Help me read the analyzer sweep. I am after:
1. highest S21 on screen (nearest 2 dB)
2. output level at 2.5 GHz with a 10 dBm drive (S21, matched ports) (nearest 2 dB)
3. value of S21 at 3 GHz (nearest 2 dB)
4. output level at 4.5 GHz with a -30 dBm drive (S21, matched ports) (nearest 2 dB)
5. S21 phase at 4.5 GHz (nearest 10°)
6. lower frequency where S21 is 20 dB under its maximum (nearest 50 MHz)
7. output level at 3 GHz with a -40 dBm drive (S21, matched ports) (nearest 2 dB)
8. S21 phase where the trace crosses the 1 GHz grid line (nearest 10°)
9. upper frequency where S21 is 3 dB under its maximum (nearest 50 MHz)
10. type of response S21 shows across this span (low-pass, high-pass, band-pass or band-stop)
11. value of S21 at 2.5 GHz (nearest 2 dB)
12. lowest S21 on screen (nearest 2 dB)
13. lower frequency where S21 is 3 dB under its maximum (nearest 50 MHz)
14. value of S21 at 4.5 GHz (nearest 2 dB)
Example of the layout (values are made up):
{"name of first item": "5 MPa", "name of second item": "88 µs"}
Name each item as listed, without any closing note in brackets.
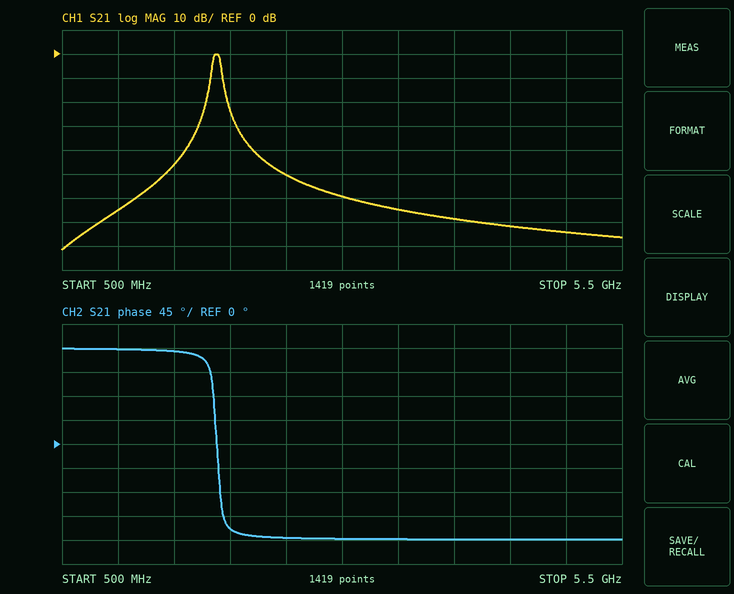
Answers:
{"highest S21 on screen": "0 dB", "output level at 2.5 GHz with a 10 dBm drive (S21, matched ports)": "-40 dBm", "value of S21 at 3 GHz": "-60 dB", "output level at 4.5 GHz with a -30 dBm drive (S21, matched ports)": "-102 dBm", "S21 phase at 4.5 GHz": "-180°", "lower frequency where S21 is 20 dB under its maximum": "1.80 GHz", "output level at 3 GHz with a -40 dBm drive (S21, matched ports)": "-100 dBm", "S21 phase where the trace crosses the 1 GHz grid line": "180°", "upper frequency where S21 is 3 dB under its maximum": "1.90 GHz", "type of response S21 shows across this span": "band-pass", "value of S21 at 2.5 GHz": "-50 dB", "lowest S21 on screen": "-82 dB", "lower frequency where S21 is 3 dB under its maximum": "1.85 GHz", "value of S21 at 4.5 GHz": "-72 dB"}
